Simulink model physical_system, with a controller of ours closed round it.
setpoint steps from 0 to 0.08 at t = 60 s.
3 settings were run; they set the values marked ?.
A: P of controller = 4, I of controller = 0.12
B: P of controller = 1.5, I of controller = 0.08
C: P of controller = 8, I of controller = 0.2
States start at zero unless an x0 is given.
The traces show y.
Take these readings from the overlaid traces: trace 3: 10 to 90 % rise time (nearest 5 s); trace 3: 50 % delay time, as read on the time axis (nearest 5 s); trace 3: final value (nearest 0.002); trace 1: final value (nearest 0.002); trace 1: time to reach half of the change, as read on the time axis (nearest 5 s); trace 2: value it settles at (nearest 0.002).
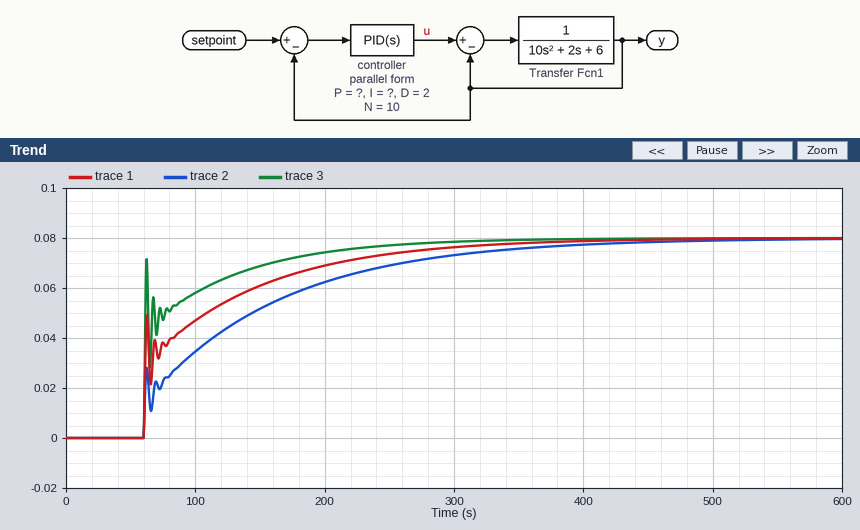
115 s
60 s
0.080
0.080
60 s
0.080
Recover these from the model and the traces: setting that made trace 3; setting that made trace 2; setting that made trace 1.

C
B
A
